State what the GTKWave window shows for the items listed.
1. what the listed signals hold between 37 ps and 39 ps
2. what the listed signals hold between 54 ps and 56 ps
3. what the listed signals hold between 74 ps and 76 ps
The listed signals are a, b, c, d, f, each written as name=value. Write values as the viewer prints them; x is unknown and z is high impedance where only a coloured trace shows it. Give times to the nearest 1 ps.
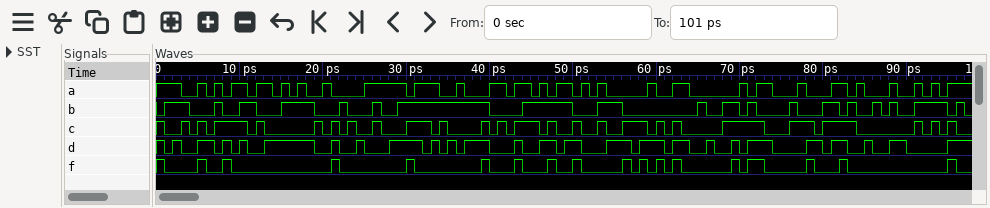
a=0, b=1, c=0, d=1, f=0
a=0, b=1, c=0, d=1, f=0
a=0, b=0, c=0, d=0, f=0
